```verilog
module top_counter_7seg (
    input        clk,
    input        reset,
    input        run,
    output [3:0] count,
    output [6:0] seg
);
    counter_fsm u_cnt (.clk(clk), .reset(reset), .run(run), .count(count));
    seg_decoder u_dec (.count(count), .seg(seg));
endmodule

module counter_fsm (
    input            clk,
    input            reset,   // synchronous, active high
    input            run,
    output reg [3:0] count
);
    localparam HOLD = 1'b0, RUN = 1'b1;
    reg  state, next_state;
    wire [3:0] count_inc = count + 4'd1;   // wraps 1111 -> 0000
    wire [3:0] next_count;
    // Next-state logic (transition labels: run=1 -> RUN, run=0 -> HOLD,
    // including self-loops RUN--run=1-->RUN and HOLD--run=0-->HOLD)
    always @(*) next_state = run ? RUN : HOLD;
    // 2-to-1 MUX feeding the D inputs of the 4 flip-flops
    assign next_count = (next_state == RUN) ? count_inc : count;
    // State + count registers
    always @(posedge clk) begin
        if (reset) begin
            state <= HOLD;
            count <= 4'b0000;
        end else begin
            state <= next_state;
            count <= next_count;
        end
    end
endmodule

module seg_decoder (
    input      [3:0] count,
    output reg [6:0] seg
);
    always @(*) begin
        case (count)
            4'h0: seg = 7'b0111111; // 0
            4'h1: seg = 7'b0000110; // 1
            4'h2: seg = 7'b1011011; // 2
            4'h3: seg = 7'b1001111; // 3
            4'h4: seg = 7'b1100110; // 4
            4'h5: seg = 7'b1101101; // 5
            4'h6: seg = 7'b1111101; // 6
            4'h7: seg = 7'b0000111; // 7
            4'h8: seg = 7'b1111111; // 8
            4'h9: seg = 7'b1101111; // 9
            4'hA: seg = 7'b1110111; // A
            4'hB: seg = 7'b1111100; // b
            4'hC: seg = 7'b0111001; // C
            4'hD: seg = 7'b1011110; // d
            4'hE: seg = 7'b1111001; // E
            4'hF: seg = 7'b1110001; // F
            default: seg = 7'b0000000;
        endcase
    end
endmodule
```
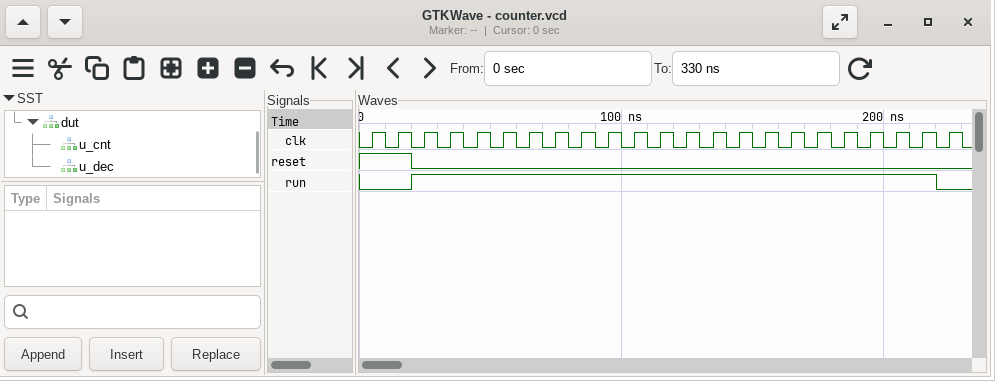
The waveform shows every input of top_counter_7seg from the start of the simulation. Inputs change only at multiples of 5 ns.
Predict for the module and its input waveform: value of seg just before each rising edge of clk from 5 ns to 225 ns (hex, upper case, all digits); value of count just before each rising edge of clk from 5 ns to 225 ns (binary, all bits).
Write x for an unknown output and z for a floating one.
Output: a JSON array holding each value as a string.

["x, 3F, 3F, 06, 5B, 4F, 66, 6D, 7D, 07, 7F, 6F, 77, 7C, 39, 5E, 79, 71, 3F, 06, 5B, 4F, 66", "x, 0000, 0000, 0001, 0010, 0011, 0100, 0101, 0110, 0111, 1000, 1001, 1010, 1011, 1100, 1101, 1110, 1111, 0000, 0001, 0010, 0011, 0100"]
